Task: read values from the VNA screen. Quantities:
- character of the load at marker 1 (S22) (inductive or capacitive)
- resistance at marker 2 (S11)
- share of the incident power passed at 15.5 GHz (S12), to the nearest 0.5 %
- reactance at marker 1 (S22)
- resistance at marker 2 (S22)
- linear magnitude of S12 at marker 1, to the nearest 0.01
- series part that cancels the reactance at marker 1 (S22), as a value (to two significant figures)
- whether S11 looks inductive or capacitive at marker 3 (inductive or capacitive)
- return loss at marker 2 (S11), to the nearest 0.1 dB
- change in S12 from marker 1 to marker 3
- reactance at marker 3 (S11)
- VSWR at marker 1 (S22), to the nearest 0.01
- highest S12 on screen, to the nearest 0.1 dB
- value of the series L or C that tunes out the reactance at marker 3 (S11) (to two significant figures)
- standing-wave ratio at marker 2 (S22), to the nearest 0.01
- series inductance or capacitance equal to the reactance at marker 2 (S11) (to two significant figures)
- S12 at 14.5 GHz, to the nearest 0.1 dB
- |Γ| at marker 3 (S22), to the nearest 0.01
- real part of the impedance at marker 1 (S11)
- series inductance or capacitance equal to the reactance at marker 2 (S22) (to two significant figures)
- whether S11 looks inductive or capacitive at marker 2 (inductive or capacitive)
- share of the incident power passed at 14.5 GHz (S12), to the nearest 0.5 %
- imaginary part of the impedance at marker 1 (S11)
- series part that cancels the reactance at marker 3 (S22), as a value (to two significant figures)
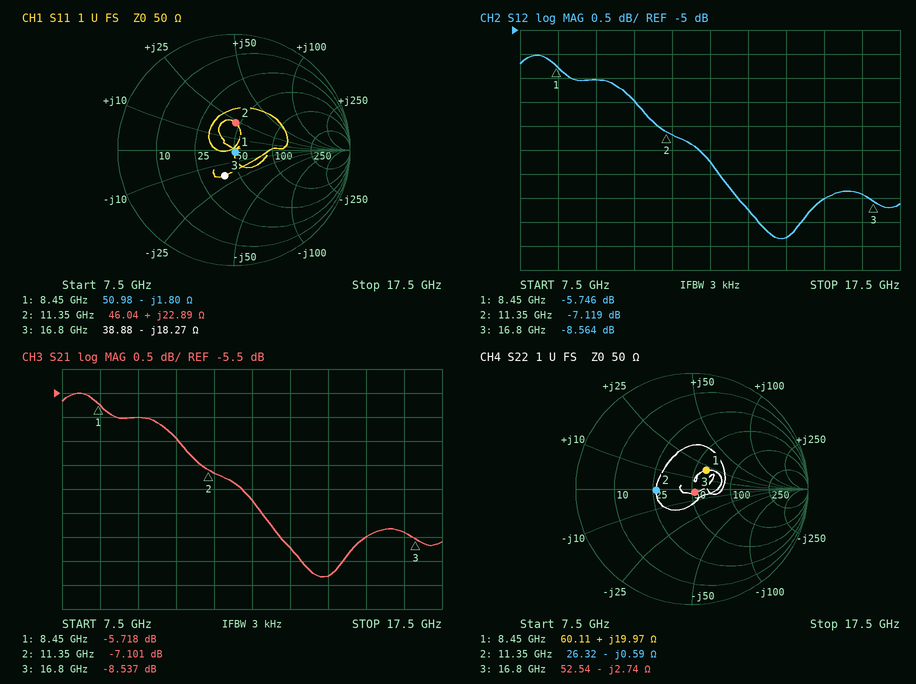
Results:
inductive
46.04 Ω
14.0 %
+19.97 Ω
26.32 Ω
0.52
940 fF
capacitive
12.6 dB
-2.818 dB
-18.27 Ω
1.50
-5.5 dB
170 pH
1.90
320 pH
-9.3 dB
0.04
50.98 Ω
24 pF
inductive
11.5 %
-1.80 Ω
26 pH
